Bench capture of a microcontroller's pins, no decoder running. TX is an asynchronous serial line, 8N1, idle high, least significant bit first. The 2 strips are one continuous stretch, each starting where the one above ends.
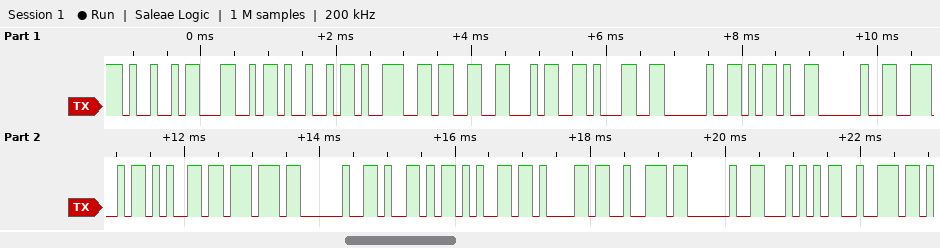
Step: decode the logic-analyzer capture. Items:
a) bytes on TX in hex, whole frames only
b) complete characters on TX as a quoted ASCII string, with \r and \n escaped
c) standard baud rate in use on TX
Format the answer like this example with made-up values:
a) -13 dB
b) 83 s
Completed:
a) 49 4C 49 39 33 34 31 20 2D 20 4E 65 77 20 59 65 61 72 20 54 72
b) "ILI9341 - New Year Tr"
c) 9600 baud
